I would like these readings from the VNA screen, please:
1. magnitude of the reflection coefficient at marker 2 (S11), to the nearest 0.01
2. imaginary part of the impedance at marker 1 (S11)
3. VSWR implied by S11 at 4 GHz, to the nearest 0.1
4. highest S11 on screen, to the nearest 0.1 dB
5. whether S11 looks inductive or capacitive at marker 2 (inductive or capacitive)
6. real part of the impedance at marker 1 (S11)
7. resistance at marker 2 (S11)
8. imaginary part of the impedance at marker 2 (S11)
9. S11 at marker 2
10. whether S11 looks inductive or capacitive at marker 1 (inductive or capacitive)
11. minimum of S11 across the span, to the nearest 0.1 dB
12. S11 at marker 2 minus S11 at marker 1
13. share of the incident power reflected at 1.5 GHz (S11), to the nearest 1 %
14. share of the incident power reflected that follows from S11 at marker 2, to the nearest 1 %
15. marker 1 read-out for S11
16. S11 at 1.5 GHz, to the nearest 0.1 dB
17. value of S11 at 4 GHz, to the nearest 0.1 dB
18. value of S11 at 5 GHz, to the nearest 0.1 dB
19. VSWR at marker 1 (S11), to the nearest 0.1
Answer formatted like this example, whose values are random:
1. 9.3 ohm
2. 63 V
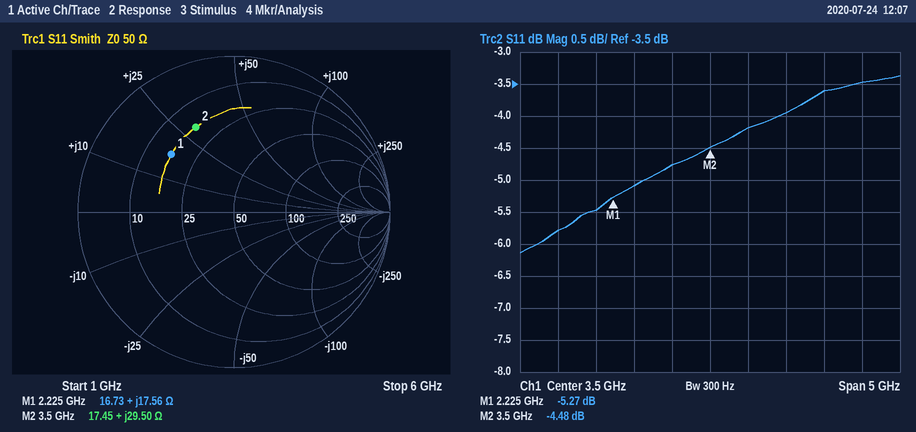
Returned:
1. 0.60
2. +17.56 Ω
3. 4.2
4. -3.4 dB
5. inductive
6. 16.73 Ω
7. 17.45 Ω
8. +29.50 Ω
9. -4.48 dB
10. inductive
11. -6.1 dB
12. 0.79 dB
13. 26 %
14. 36 %
15. -5.27 dB
16. -5.8 dB
17. -4.2 dB
18. -3.6 dB
19. 3.4
